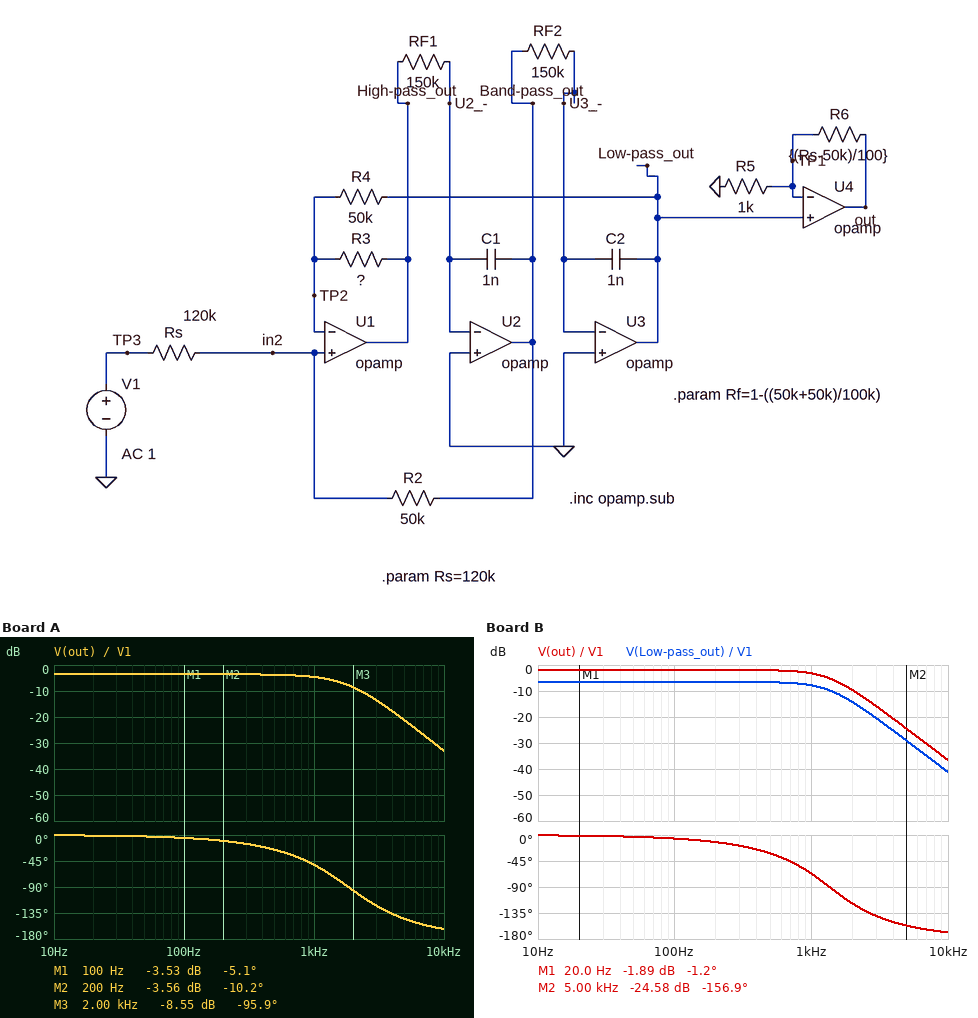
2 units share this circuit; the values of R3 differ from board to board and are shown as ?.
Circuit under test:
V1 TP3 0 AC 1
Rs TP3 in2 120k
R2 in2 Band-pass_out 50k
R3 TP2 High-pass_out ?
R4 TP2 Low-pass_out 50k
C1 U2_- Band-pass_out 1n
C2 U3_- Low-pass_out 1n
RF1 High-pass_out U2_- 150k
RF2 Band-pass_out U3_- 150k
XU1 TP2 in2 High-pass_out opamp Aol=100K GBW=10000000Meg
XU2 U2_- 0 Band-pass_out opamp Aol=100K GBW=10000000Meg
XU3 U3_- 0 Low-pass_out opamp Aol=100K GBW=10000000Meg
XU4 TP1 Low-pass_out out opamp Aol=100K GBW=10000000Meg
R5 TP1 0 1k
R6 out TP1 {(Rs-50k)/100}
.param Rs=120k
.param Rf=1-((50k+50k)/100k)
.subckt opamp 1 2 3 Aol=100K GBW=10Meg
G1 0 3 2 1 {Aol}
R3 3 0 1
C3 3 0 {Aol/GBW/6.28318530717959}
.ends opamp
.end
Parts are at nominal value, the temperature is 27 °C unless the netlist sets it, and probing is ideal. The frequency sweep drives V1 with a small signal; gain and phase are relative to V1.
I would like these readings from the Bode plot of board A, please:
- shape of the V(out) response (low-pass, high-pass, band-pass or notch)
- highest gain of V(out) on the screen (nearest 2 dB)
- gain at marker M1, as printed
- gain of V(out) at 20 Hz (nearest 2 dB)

low-pass
-4 dB
-3.53 dB
-4 dB
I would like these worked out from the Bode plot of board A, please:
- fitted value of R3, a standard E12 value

150 kΩ
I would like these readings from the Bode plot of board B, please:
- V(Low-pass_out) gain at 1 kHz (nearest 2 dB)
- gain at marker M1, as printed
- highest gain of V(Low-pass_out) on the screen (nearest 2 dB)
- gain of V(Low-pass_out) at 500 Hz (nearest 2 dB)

-8 dB
-1.89 dB
-6 dB
-6 dB
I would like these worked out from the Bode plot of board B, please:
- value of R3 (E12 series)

82 kΩ
